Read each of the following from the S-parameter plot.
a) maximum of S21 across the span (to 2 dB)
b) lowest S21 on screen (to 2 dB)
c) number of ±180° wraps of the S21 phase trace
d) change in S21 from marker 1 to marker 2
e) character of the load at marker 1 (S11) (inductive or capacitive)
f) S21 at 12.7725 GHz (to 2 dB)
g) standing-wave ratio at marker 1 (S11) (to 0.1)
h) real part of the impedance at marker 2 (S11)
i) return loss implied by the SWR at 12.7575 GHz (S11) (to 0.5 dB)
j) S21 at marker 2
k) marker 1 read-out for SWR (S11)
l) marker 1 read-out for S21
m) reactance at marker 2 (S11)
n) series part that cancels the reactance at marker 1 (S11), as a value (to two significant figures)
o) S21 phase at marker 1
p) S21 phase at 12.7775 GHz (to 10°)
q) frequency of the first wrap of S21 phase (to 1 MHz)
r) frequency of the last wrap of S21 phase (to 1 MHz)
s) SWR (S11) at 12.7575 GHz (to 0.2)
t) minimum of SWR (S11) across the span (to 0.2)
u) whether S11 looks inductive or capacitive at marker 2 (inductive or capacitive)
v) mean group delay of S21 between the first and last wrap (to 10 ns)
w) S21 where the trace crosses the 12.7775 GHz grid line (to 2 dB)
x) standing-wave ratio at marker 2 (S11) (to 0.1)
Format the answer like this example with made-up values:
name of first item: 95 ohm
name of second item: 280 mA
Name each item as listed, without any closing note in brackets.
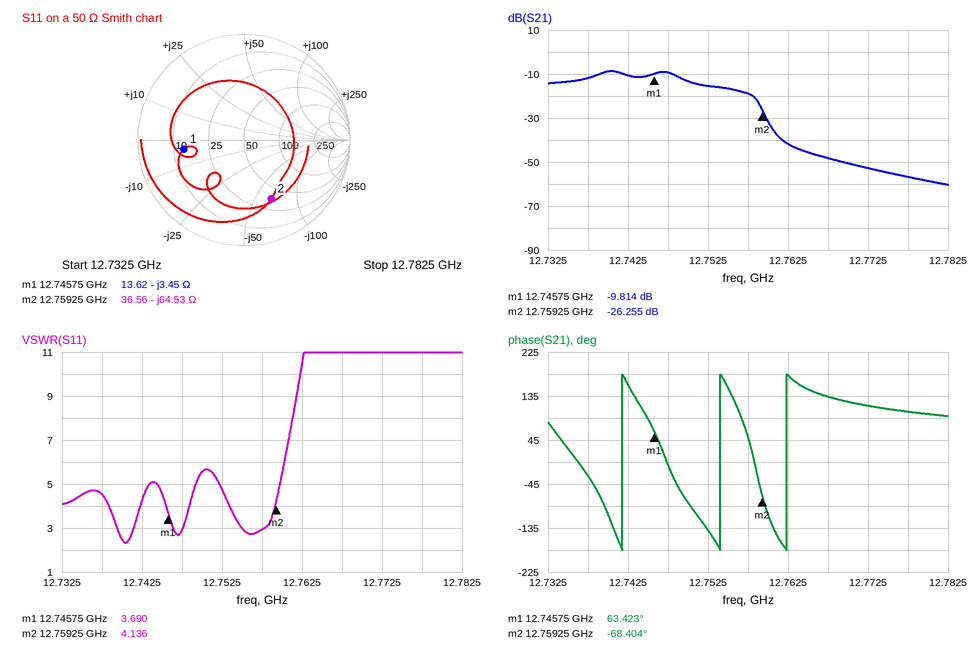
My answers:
maximum of S21 across the span: -8 dB
lowest S21 on screen: -60 dB
number of ±180° wraps of the S21 phase trace: 3
change in S21 from marker 1 to marker 2: -16.441 dB
character of the load at marker 1 (S11): capacitive
S21 at 12.7725 GHz: -52 dB
standing-wave ratio at marker 1 (S11): 3.7
real part of the impedance at marker 2: 36.56 Ω
return loss implied by the SWR at 12.7575 GHz (S11): 6.0 dB
S21 at marker 2: -26.255 dB
marker 1 read-out for SWR: 3.690
marker 1 read-out for S21: -9.814 dB
reactance at marker 2: -64.53 Ω
series part that cancels the reactance at marker 1 (S11), as a value: 43 pH
S21 phase at marker 1: 63.423°
S21 phase at 12.7775 GHz: 100°
frequency of the first wrap of S21 phase: 12.742 GHz
frequency of the last wrap of S21 phase: 12.762 GHz
SWR (S11) at 12.7575 GHz: 3.0
minimum of SWR (S11) across the span: 2.4
whether S11 looks inductive or capacitive at marker 2: capacitive
mean group delay of S21 between the first and last wrap: 100 ns
S21 where the trace crosses the 12.7775 GHz grid line: -56 dB
standing-wave ratio at marker 2 (S11): 4.1
